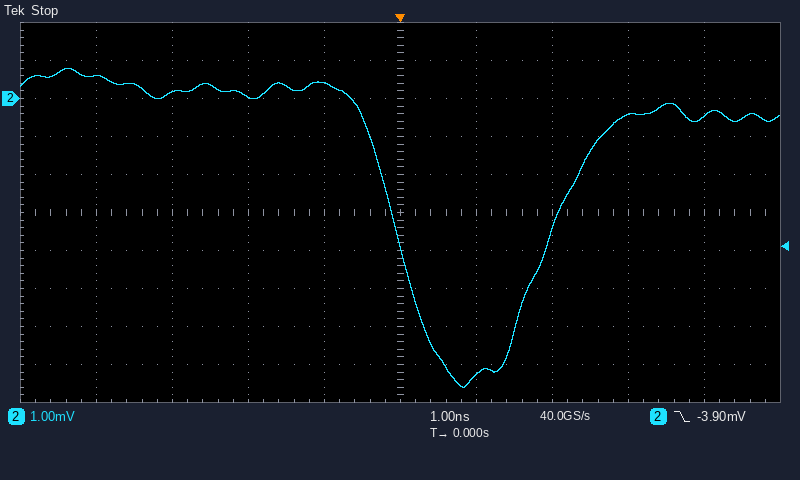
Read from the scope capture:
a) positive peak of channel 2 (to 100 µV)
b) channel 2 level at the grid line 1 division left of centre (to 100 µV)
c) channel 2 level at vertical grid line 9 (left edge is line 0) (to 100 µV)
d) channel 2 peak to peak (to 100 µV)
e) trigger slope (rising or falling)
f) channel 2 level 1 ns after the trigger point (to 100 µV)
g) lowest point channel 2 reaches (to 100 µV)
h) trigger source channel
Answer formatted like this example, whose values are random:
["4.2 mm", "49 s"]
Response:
["800 µV", "400 µV", "-500 µV", "8.4 mV", "falling", "-7.3 mV", "-7.6 mV", "channel 2"]
